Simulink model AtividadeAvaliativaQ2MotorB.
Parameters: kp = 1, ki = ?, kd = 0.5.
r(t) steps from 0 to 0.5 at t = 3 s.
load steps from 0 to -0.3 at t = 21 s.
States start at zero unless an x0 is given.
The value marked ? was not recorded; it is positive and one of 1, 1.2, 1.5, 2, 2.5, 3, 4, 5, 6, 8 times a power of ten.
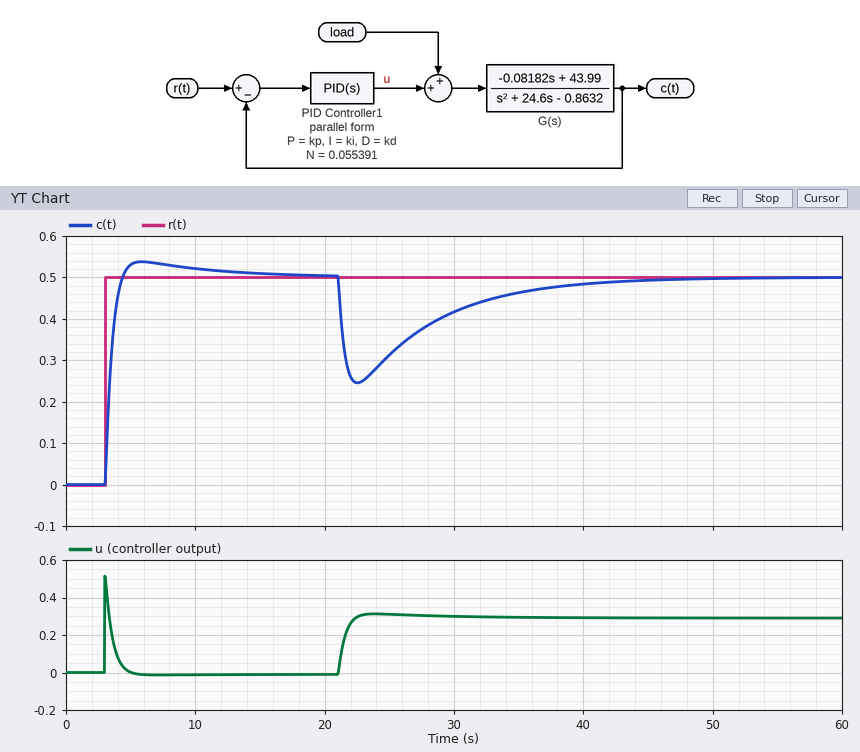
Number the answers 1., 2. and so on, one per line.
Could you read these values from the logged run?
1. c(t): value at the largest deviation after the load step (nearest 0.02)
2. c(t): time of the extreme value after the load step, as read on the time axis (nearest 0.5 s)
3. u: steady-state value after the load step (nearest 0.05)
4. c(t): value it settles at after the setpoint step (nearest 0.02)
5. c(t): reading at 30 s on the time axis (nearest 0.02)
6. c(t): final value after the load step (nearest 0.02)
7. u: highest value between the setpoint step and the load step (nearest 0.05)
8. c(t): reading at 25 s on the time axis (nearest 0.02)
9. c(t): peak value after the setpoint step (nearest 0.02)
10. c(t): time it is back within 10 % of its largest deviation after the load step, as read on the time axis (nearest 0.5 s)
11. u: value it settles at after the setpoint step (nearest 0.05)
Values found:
1. 0.24
2. 22.5 s
3. 0.30
4. 0.50
5. 0.42
6. 0.50
7. 0.50
8. 0.32
9. 0.54
10. 37.0 s
11. 0.00
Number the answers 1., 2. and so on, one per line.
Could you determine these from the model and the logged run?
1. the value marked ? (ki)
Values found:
1. 0.15
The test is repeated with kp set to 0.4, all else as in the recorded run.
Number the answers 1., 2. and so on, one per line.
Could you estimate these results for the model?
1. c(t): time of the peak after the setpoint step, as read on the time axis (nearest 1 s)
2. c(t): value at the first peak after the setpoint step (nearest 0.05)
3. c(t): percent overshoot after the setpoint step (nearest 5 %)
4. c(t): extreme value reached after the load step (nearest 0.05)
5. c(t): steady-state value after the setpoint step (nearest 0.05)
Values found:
1. 7 s
2. 0.60
3. 25 %
4. 0.00
5. 0.50
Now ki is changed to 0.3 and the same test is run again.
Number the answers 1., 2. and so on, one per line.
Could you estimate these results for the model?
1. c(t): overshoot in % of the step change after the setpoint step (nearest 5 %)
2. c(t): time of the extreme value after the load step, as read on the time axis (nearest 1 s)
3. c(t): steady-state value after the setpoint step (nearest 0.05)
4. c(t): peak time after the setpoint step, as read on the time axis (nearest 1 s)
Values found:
1. 10 %
2. 22 s
3. 0.50
4. 5 s
